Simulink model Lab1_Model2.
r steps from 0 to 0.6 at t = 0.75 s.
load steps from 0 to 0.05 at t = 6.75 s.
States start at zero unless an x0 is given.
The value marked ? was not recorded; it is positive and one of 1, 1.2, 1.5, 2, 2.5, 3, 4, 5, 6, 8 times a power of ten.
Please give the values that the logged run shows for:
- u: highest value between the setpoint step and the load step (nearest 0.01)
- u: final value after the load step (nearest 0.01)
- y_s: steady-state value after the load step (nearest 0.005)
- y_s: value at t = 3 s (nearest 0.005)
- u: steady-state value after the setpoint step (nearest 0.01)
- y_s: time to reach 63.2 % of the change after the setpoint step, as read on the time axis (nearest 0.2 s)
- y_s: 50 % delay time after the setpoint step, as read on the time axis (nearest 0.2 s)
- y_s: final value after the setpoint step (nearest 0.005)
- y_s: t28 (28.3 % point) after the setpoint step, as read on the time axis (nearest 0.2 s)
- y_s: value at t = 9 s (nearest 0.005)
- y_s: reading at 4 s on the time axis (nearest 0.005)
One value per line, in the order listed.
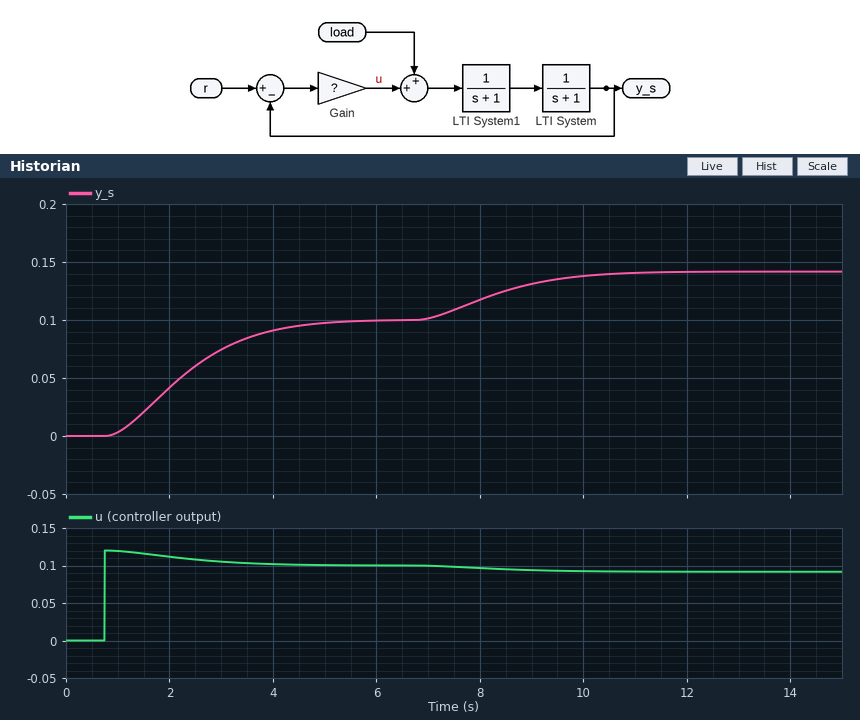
0.12
0.09
0.140
0.075
0.10
2.6 s
2.2 s
0.100
1.6 s
0.130
0.090
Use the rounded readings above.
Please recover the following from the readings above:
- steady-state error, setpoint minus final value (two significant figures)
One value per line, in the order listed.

0.50
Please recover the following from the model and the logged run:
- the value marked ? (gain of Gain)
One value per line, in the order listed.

0.2
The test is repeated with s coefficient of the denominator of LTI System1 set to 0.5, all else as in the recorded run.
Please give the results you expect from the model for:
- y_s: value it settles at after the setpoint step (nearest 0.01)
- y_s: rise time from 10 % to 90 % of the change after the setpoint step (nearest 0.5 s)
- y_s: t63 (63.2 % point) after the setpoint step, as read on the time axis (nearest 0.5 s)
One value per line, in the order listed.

0.10
2.0 s
2.0 s
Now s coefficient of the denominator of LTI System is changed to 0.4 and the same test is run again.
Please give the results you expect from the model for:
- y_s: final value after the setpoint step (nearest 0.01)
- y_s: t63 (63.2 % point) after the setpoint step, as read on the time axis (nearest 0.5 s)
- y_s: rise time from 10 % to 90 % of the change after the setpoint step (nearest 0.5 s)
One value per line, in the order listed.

0.10
2.0 s
2.0 s
